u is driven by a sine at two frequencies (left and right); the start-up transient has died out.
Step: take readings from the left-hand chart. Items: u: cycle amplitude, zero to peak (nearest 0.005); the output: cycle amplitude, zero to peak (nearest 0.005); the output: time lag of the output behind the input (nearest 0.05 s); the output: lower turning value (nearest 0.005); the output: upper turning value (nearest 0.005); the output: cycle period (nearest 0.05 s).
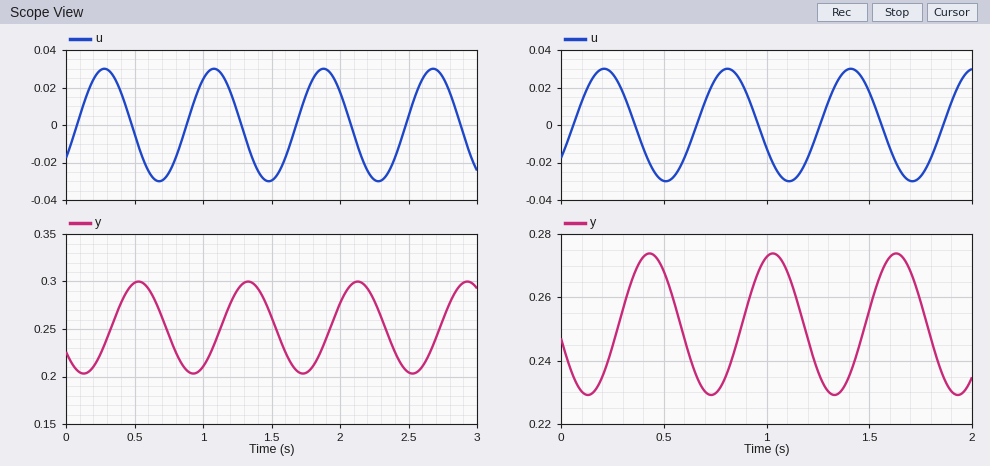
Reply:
0.030
0.050
0.25 s
0.205
0.300
0.80 s
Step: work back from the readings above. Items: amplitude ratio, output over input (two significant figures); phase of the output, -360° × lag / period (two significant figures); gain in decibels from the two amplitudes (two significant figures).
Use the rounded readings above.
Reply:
1.7
-110°
4.4 dB
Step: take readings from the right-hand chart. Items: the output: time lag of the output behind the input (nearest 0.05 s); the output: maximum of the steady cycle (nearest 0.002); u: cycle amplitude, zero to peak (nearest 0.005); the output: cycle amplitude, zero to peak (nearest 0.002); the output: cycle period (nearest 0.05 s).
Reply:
0.20 s
0.274
0.030
0.022
0.60 s
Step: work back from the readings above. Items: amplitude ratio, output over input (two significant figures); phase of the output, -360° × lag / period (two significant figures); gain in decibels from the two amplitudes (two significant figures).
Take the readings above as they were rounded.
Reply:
0.73
-120°
-2.7 dB
